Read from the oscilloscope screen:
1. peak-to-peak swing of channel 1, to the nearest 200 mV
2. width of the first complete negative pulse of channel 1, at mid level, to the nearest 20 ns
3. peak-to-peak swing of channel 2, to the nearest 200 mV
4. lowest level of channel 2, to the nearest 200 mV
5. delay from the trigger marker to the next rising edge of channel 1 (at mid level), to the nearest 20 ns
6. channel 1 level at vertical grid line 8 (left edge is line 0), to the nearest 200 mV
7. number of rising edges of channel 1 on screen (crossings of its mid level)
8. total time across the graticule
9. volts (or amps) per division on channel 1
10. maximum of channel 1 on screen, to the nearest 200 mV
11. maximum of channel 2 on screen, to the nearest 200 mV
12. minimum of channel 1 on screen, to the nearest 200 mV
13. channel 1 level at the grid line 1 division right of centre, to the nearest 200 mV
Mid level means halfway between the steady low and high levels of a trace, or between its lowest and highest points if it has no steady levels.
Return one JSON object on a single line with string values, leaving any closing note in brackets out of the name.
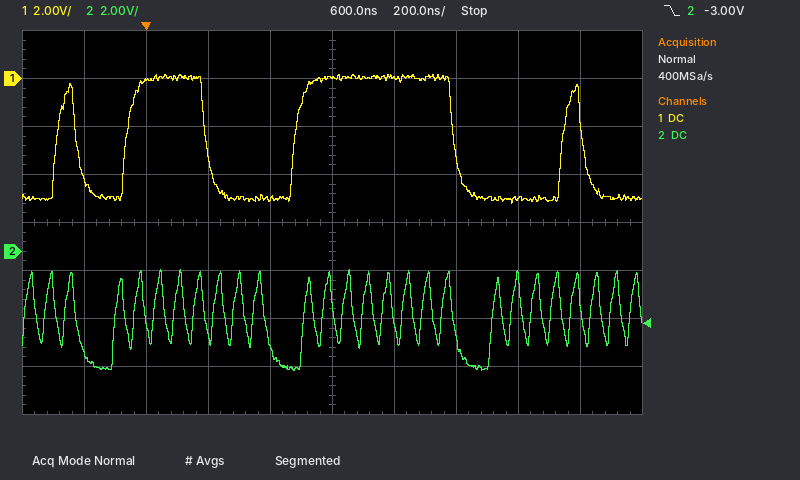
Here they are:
{"peak-to-peak swing of channel 1, to the nearest 200 mV": "5.4 V", "width of the first complete negative pulse of channel 1, at mid level, to the nearest 20 ns": "160 ns", "peak-to-peak swing of channel 2, to the nearest 200 mV": "4.2 V", "lowest level of channel 2, to the nearest 200 mV": "-5.0 V", "delay from the trigger marker to the next rising edge of channel 1 (at mid level), to the nearest 20 ns": "480 ns", "channel 1 level at vertical grid line 8 (left edge is line 0), to the nearest 200 mV": "-5.0 V", "number of rising edges of channel 1 on screen": "4", "total time across the graticule": "2 µs", "volts (or amps) per division on channel 1": "2 V", "maximum of channel 1 on screen, to the nearest 200 mV": "200 mV", "maximum of channel 2 on screen, to the nearest 200 mV": "-800 mV", "minimum of channel 1 on screen, to the nearest 200 mV": "-5.2 V", "channel 1 level at the grid line 1 division right of centre, to the nearest 200 mV": "0.0 V"}
